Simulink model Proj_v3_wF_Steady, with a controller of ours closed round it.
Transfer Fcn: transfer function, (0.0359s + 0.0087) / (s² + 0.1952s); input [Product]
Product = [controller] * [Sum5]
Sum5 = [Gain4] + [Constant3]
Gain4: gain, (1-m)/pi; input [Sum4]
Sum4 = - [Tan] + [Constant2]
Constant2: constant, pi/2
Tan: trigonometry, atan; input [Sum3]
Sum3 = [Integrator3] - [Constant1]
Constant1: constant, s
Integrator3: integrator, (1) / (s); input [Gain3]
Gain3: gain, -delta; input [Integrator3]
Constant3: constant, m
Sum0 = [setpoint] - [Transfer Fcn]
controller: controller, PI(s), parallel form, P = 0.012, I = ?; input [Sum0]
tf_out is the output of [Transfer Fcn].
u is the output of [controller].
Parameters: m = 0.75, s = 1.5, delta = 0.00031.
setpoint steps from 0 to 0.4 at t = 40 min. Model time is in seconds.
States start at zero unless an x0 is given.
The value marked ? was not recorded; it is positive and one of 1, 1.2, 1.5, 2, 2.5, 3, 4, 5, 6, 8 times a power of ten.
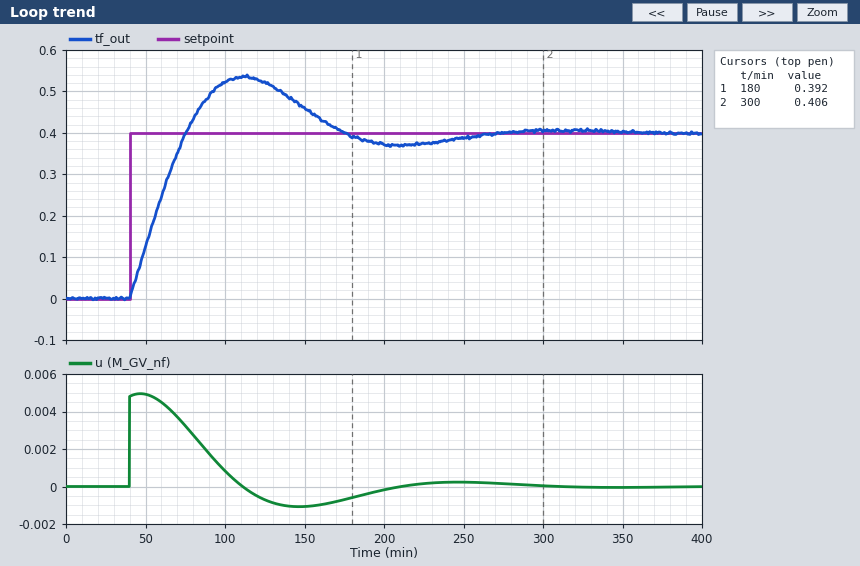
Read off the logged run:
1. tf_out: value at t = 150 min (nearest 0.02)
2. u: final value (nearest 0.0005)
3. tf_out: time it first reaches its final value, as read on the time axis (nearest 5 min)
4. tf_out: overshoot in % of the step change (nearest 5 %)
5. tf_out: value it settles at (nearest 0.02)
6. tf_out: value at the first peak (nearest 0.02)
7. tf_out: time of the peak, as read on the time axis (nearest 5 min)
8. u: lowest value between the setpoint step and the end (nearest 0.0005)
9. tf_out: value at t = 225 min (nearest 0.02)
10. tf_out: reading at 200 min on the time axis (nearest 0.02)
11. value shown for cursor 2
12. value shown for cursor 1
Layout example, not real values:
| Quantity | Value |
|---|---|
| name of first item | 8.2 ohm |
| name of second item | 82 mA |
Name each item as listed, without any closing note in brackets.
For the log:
| Quantity | Value |
|---|---|
| tf_out: value at t = 150 min | 0.46 |
| u: final value | 0.0000 |
| tf_out: time it first reaches its final value, as read on the time axis | 75 min |
| tf_out: overshoot in % of the step change | 35 % |
| tf_out: value it settles at | 0.40 |
| tf_out: value at the first peak | 0.54 |
| tf_out: time of the peak, as read on the time axis | 110 min |
| u: lowest value between the setpoint step and the end | -0.0010 |
| tf_out: value at t = 225 min | 0.38 |
| tf_out: reading at 200 min on the time axis | 0.38 |
| value shown for cursor 2 | 0.406 |
| value shown for cursor 1 | 0.392 |
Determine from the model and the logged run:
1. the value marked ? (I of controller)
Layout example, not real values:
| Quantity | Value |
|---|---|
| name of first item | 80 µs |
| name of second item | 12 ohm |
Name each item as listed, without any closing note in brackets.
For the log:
| Quantity | Value |
|---|---|
| the value marked ? | 8e-06 |
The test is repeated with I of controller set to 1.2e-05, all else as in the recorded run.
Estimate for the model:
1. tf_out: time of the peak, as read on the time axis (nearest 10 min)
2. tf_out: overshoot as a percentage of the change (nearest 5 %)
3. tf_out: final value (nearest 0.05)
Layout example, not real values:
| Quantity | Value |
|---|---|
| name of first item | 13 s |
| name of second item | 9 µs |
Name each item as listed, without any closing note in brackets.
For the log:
| Quantity | Value |
|---|---|
| tf_out: time of the peak, as read on the time axis | 100 min |
| tf_out: overshoot as a percentage of the change | 40 % |
| tf_out: final value | 0.40 |
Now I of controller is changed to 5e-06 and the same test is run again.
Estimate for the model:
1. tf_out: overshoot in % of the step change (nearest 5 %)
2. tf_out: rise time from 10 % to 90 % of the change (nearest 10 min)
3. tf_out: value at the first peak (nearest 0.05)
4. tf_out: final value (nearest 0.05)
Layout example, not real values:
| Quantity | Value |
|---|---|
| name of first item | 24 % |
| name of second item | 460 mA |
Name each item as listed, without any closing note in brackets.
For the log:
| Quantity | Value |
|---|---|
| tf_out: overshoot in % of the step change | 25 % |
| tf_out: rise time from 10 % to 90 % of the change | 30 min |
| tf_out: value at the first peak | 0.50 |
| tf_out: final value | 0.40 |
